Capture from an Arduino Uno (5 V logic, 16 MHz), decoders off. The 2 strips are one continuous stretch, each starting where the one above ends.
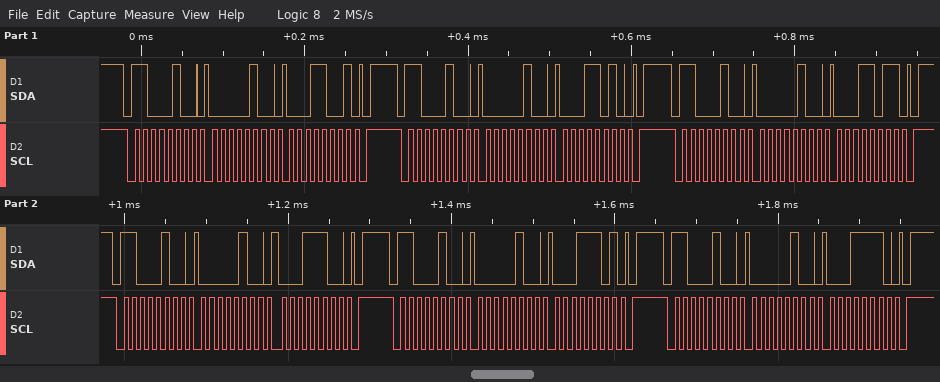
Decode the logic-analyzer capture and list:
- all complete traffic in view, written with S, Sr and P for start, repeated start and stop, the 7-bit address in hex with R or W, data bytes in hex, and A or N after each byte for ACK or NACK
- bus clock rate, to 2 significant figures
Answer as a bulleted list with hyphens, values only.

- S 62W A 04 A 19 A P S 62W A 04 A 1A A P S 62W A 04 A 1B A P S 62W A 04 A 1C A P S 62W A 04 A 1D A P S 62W A 04 A 1E A P
- 100 kHz
